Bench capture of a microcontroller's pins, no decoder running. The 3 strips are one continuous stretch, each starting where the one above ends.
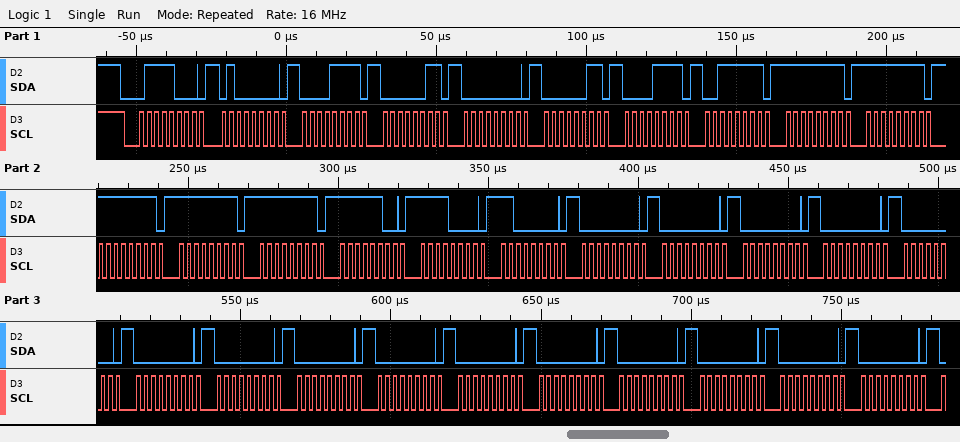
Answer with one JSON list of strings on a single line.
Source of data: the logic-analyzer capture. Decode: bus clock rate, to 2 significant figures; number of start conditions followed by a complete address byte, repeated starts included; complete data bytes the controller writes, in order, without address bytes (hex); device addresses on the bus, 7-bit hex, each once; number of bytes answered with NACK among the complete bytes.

["400 kHz", "1", "40 0F 03 00 03 0F 3F FF FF FF FF FF FC F0 C0 00 00 00 00 00 00 00 00 00 00 00 00 00 00 00", "0x3C", "0"]
